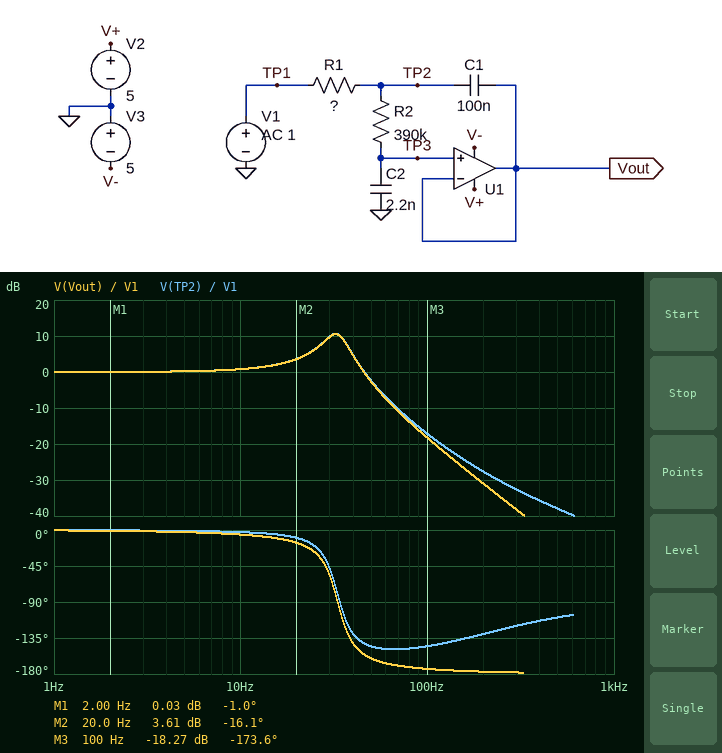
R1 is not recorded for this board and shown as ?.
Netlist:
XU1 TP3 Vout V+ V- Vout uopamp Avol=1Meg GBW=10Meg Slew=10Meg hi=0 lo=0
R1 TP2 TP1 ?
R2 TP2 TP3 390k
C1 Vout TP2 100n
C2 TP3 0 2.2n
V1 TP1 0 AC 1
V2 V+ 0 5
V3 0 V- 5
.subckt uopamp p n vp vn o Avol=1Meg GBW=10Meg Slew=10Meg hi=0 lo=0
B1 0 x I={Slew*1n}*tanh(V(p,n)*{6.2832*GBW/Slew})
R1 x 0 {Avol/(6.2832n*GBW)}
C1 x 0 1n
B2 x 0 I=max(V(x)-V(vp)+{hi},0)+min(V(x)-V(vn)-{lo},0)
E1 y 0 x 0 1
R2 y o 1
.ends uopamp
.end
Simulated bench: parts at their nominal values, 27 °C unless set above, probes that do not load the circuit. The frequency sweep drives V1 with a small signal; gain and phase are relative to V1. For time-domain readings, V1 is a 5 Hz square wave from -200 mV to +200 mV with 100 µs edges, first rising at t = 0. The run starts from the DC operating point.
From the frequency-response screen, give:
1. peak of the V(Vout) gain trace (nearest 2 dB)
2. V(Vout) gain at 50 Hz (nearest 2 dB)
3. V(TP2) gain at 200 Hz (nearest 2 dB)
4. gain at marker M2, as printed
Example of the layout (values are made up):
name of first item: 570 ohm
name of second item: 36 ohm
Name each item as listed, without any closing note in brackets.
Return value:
peak of the V(Vout) gain trace: 10 dB
V(Vout) gain at 50 Hz: -2 dB
V(TP2) gain at 200 Hz: -28 dB
gain at marker M2, as printed: 3.61 dB
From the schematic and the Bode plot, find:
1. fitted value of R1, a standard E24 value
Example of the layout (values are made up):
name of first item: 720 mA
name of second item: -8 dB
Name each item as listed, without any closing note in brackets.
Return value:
fitted value of R1, a standard E24 value: 270 kΩ
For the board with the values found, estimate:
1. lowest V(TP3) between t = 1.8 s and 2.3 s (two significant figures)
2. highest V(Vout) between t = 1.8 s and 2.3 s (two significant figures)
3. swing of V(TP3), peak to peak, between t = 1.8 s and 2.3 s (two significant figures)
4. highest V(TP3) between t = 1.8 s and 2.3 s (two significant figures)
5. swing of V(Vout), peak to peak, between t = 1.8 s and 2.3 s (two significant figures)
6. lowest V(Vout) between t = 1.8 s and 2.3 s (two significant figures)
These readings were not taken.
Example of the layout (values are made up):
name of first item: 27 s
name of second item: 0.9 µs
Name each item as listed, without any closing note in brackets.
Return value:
lowest V(TP3) between t = 1.8 s and 2.3 s: -450 mV
highest V(Vout) between t = 1.8 s and 2.3 s: 450 mV
swing of V(TP3), peak to peak, between t = 1.8 s and 2.3 s: 890 mV
highest V(TP3) between t = 1.8 s and 2.3 s: 450 mV
swing of V(Vout), peak to peak, between t = 1.8 s and 2.3 s: 890 mV
lowest V(Vout) between t = 1.8 s and 2.3 s: -450 mV
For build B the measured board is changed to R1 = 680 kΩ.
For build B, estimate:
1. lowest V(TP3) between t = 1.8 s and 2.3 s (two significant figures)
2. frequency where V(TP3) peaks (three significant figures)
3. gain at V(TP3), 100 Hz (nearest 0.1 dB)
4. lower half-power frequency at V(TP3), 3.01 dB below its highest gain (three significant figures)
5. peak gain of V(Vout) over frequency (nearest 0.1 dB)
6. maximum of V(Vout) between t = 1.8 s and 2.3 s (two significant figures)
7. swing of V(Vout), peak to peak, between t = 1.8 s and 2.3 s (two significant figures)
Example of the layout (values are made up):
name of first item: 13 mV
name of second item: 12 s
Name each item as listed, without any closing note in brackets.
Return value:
lowest V(TP3) between t = 1.8 s and 2.3 s: -420 mV
frequency where V(TP3) peaks: 20.3 Hz
gain at V(TP3), 100 Hz: -26.9 dB
lower half-power frequency at V(TP3), 3.01 dB below its highest gain: 16.8 Hz
peak gain of V(Vout) over frequency: 10.3 dB
maximum of V(Vout) between t = 1.8 s and 2.3 s: 420 mV
swing of V(Vout), peak to peak, between t = 1.8 s and 2.3 s: 830 mV
